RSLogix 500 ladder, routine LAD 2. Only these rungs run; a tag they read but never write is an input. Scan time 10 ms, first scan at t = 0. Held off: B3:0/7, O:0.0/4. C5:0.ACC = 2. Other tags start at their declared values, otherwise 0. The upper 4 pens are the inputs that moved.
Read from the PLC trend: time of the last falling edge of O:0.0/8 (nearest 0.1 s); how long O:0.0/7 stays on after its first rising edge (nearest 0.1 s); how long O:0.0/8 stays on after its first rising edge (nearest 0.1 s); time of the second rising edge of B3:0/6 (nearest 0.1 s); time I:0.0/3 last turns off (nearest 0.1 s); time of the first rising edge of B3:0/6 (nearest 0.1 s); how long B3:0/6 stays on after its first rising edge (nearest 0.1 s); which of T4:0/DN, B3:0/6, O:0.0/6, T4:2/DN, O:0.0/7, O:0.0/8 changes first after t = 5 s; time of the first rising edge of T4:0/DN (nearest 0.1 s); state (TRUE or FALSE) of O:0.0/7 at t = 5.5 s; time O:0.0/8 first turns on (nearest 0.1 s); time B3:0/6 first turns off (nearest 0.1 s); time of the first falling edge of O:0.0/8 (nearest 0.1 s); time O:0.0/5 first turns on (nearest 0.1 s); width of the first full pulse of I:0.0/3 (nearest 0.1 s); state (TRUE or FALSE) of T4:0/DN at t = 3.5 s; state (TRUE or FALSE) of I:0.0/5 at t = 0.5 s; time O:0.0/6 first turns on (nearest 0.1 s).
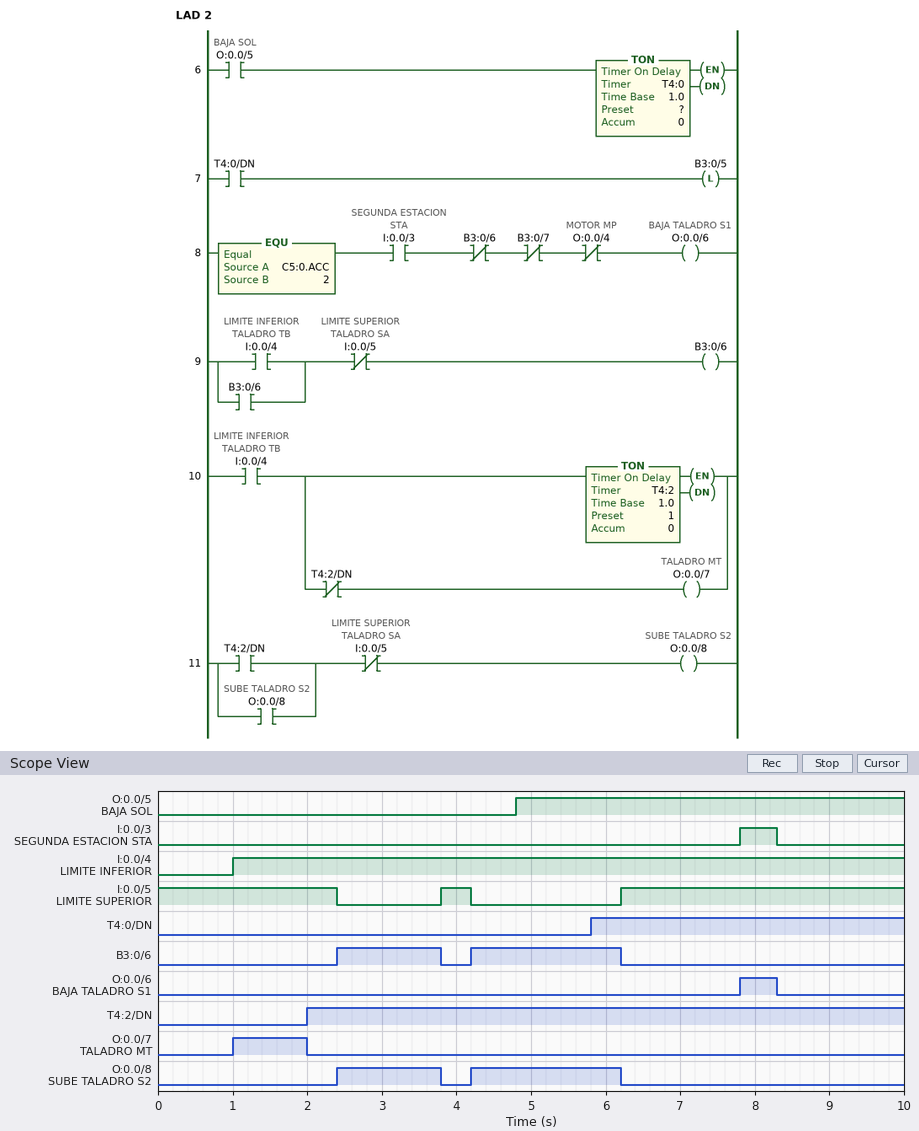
6.2 s
1.0 s
1.4 s
4.2 s
8.3 s
2.4 s
1.4 s
T4:0/DN
5.8 s
FALSE
2.4 s
3.8 s
3.8 s
4.8 s
0.5 s
FALSE
TRUE
7.8 s
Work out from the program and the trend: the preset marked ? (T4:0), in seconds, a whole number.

1 s
